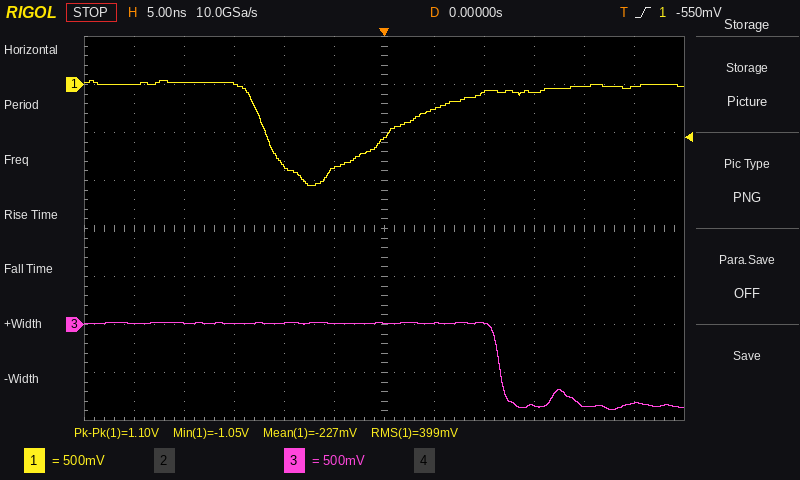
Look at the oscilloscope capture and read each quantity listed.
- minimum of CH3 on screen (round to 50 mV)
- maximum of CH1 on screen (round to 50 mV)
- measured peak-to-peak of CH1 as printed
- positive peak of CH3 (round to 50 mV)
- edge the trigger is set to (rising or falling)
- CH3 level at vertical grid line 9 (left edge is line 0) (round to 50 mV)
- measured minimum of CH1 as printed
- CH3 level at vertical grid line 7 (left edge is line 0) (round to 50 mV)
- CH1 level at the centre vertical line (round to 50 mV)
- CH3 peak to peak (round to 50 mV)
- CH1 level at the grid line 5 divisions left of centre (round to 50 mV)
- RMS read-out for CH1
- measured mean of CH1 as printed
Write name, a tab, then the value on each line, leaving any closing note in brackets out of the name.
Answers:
minimum of CH3 on screen	-900 mV
maximum of CH1 on screen	50 mV
measured peak-to-peak of CH1 as printed	1.10 V
positive peak of CH3	0 mV
edge the trigger is set to	rising
CH3 level at vertical grid line 9 (left edge is line 0)	-850 mV
measured minimum of CH1 as printed	-1.05 V
CH3 level at vertical grid line 7 (left edge is line 0)	0 mV
CH1 level at the centre vertical line	-550 mV
CH3 peak to peak	900 mV
CH1 level at the grid line 5 divisions left of centre	0 mV
RMS read-out for CH1	399 mV
measured mean of CH1 as printed	-227 mV
